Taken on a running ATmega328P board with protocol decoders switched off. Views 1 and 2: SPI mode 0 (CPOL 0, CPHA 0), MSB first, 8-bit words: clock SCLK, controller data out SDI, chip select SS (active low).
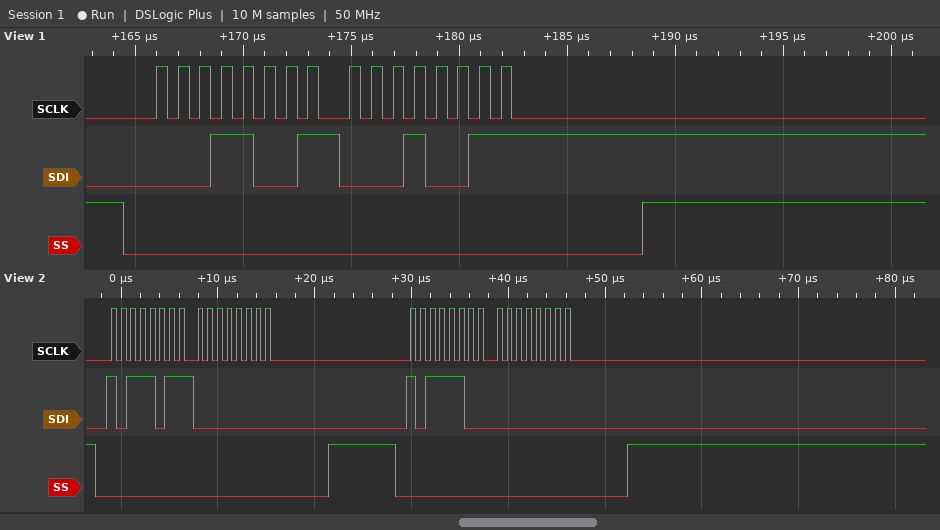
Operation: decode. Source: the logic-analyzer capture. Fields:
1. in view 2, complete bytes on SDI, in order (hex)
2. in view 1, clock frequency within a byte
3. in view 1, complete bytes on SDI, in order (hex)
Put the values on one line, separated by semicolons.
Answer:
0xBB 0x00 0xBC 0x00; 1 MHz; 0x19 0x13
